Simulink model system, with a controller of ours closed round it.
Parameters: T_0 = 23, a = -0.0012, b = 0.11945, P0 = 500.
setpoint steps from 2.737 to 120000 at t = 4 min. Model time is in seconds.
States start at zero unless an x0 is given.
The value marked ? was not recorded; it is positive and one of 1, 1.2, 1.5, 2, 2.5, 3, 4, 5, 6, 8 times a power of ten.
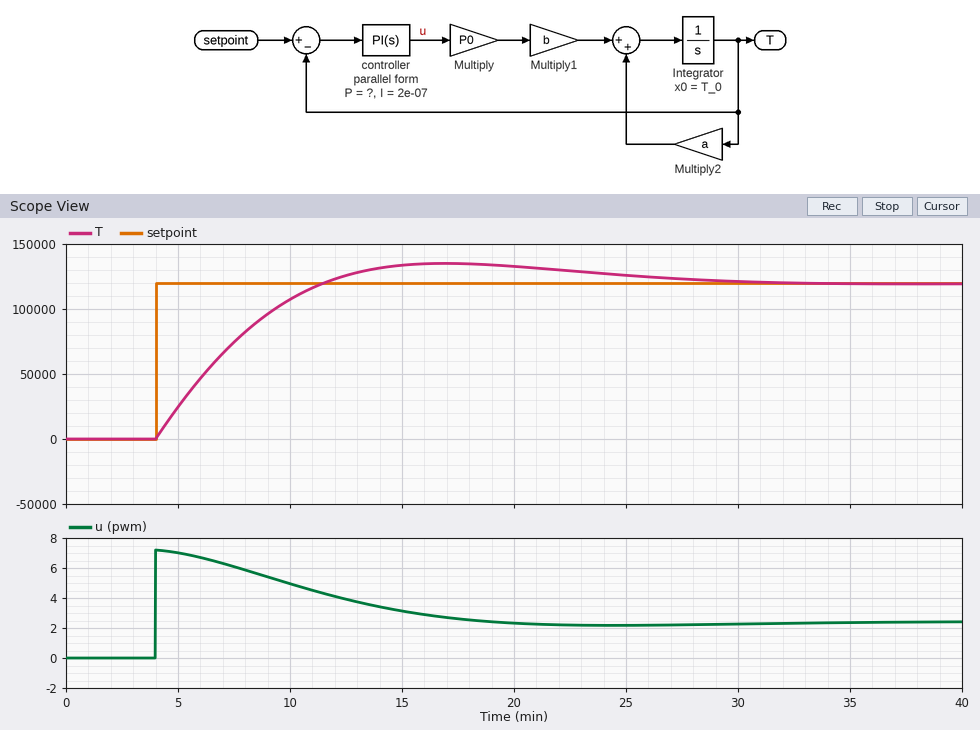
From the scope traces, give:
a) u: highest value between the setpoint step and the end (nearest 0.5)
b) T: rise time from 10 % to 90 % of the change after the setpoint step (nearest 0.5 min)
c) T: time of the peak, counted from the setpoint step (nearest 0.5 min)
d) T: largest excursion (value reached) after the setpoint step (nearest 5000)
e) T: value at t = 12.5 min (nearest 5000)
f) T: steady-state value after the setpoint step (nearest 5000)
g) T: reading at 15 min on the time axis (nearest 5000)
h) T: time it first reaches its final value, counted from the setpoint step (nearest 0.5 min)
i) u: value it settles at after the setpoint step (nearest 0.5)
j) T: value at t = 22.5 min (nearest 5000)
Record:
7.0
5.5 min
13.0 min
135000
125000
120000
135000
7.5 min
2.5
130000
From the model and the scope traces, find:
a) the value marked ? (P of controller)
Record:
6e-05
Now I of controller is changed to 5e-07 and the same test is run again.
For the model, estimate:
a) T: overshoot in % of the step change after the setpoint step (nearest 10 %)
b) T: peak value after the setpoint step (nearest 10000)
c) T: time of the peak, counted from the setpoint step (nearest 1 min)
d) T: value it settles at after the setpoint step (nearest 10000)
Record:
30 %
150000
8 min
120000
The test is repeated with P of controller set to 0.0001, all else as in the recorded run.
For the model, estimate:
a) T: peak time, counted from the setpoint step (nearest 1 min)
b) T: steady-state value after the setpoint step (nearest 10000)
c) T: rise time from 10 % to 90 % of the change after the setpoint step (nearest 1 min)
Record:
12 min
120000
5 min
